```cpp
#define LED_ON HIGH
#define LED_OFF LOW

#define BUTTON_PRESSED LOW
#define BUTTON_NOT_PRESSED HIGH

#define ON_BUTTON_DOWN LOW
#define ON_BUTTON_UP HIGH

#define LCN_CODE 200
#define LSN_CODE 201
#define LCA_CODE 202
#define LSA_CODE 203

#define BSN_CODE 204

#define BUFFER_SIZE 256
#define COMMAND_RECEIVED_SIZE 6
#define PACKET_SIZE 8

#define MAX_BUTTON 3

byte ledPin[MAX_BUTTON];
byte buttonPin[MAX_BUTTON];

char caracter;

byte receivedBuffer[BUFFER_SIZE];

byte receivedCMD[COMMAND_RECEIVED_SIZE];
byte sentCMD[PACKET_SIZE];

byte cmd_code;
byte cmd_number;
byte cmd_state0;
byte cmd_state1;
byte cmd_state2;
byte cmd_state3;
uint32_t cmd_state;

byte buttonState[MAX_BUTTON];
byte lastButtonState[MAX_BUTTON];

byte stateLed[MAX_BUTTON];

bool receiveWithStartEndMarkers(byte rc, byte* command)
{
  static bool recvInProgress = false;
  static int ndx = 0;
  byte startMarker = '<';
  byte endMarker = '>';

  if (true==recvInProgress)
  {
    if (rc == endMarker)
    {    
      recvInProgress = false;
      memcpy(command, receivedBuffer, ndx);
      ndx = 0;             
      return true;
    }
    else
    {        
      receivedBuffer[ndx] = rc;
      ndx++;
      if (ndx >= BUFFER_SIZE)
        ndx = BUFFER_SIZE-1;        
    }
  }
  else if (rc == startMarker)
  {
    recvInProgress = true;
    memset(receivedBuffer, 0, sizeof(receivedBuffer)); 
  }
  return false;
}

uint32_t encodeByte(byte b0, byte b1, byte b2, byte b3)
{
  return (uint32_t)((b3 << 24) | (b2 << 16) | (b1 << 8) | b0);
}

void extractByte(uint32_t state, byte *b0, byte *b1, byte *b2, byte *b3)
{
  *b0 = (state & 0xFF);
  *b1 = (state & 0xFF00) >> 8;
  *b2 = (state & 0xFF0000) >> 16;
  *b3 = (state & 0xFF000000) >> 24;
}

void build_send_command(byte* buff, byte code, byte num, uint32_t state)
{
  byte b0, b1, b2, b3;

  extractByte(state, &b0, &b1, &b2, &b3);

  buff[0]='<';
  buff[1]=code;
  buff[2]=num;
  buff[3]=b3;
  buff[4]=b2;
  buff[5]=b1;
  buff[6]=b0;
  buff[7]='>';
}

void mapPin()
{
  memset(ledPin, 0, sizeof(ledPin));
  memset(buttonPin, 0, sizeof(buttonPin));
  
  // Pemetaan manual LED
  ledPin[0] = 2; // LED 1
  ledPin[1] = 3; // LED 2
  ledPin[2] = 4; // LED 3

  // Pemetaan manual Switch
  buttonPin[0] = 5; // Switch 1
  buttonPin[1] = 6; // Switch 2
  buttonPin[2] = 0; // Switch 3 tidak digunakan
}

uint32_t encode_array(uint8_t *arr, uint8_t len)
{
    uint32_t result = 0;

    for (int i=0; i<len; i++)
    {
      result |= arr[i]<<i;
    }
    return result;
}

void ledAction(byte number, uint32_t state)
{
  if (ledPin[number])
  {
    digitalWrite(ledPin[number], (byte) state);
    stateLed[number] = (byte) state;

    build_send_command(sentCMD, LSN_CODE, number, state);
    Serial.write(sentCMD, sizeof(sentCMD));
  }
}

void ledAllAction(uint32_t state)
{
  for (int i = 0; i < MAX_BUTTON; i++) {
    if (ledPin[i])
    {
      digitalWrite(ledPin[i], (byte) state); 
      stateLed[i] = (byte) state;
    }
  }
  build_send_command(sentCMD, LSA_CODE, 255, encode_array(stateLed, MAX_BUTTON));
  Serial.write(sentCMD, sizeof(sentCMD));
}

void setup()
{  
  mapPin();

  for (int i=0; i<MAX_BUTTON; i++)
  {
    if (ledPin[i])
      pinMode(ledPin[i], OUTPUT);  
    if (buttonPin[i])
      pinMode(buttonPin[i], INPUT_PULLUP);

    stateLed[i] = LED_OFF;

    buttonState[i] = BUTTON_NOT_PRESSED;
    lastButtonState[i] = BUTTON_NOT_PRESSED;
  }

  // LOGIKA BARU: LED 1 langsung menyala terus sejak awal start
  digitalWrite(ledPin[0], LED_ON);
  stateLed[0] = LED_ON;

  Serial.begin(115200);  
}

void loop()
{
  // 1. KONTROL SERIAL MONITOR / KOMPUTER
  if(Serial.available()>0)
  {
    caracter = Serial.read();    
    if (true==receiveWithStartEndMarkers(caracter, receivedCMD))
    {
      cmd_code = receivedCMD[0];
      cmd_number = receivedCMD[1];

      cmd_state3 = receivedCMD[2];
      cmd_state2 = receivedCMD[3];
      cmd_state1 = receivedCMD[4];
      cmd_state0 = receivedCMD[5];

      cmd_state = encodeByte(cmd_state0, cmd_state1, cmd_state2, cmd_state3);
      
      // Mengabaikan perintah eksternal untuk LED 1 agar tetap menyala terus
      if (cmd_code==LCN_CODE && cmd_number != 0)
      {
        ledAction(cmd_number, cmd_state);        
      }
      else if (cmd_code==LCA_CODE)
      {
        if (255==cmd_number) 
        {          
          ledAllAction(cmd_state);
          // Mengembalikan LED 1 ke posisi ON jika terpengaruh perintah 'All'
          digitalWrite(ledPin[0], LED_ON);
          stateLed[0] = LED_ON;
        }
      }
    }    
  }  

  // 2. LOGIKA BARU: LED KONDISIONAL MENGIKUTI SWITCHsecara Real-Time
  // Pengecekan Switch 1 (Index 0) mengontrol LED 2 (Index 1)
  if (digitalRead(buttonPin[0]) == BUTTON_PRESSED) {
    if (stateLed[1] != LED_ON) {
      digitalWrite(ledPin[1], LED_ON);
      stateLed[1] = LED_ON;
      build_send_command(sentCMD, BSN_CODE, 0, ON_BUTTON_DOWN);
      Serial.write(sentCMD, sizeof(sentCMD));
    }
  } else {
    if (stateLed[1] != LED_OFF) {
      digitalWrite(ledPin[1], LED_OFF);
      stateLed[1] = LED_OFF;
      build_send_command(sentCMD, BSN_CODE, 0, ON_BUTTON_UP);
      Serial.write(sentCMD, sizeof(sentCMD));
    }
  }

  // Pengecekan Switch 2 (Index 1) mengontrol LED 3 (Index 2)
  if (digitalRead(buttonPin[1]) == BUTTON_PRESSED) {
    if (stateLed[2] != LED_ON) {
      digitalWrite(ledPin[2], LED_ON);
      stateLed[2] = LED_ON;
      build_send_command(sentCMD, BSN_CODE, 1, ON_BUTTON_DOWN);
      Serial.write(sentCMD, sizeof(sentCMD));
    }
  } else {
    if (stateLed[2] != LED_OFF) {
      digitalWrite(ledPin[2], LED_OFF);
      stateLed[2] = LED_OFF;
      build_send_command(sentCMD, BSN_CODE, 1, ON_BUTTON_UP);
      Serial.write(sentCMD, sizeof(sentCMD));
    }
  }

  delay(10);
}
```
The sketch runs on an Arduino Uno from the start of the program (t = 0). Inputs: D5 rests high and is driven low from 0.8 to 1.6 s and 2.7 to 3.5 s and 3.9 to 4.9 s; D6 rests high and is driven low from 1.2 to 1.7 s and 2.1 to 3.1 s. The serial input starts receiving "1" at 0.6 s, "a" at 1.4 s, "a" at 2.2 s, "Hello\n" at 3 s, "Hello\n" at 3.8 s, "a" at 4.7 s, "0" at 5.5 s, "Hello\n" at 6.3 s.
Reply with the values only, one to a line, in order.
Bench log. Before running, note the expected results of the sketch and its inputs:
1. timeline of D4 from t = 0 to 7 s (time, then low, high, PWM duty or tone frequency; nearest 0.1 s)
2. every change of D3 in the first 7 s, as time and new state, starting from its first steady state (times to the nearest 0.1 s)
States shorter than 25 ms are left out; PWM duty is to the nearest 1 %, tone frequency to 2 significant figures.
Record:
0 s low; 1.2 s high; 1.7 s low; 2.1 s high; 3.1 s low
0 s low; 0.8 s high; 1.6 s low; 2.7 s high; 3.5 s low; 3.9 s high; 4.9 s low
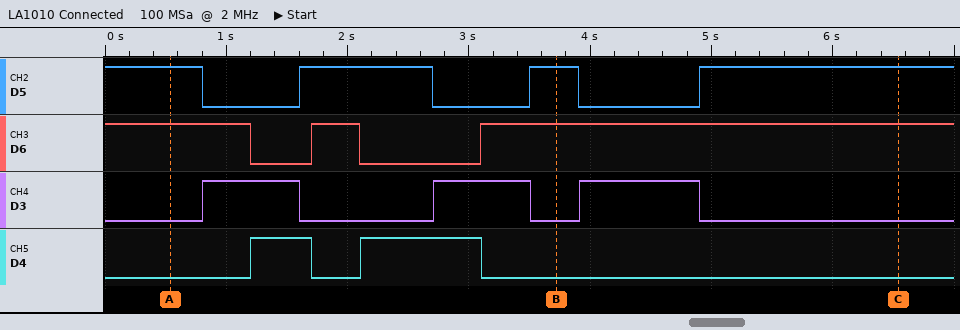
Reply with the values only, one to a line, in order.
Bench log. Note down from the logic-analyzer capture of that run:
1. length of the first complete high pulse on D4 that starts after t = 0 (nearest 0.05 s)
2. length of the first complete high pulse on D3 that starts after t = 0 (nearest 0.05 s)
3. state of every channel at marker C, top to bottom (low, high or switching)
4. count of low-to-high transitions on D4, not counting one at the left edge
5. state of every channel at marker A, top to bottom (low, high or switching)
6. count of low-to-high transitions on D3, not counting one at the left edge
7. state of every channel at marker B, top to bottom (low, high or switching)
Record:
0.50 s
0.80 s
D5 high, D6 high, D3 low, D4 low
2
D5 high, D6 high, D3 low, D4 low
3
D5 high, D6 high, D3 low, D4 low
